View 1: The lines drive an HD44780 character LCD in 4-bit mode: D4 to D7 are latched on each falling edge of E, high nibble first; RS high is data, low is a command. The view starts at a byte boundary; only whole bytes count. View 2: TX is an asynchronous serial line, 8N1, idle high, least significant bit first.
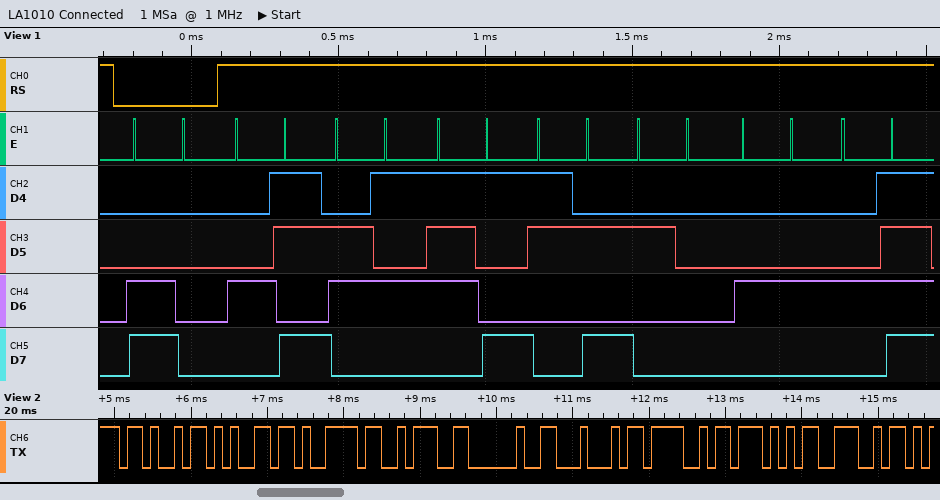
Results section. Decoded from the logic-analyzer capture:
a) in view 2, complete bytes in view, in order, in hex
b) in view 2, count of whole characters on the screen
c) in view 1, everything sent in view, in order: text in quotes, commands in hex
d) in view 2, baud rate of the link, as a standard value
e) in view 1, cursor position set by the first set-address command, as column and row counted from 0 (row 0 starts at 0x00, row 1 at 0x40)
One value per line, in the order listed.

4B 65 79 3A 20 44 4F 57 4E
9
0xC0 "Key: DO"
9600 baud
column 0, row 1
